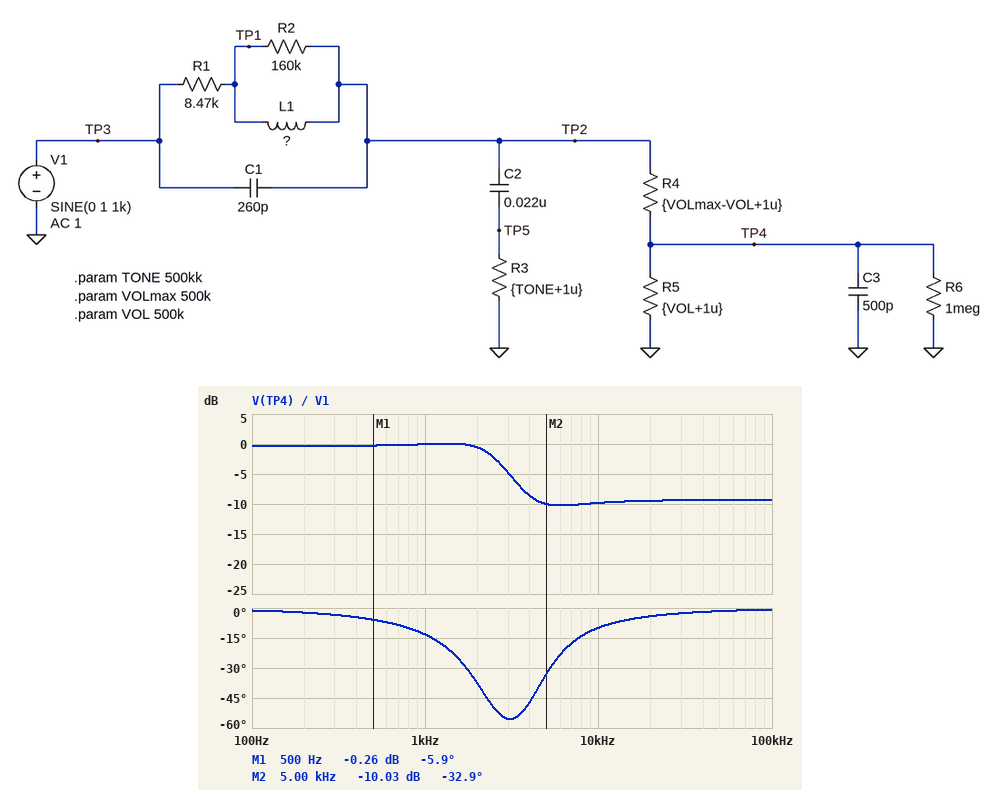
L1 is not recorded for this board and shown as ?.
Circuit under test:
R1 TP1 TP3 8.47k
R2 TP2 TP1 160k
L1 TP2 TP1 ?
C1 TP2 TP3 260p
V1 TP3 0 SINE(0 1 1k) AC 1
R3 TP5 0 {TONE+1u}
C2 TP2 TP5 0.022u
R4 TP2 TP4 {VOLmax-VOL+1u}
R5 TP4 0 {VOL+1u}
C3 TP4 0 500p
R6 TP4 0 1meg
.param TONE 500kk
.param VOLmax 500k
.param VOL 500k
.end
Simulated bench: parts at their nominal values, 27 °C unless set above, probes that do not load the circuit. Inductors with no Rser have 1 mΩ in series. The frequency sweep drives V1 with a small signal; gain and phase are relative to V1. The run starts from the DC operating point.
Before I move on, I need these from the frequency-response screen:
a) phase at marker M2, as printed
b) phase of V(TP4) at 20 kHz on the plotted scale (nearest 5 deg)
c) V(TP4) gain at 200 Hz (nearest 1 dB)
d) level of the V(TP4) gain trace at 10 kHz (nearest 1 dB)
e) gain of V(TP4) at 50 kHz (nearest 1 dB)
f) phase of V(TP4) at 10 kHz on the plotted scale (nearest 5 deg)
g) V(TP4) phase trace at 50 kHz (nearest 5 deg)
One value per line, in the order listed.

-32.9 deg
-5 deg
0 dB
-10 dB
-9 dB
-10 deg
0 deg
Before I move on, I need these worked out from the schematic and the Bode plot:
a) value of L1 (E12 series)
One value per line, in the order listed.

5.6 H
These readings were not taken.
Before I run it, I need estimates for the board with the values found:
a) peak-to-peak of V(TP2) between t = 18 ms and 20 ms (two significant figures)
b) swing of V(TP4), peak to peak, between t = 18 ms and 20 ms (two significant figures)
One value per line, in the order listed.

2.0 V
2.0 V
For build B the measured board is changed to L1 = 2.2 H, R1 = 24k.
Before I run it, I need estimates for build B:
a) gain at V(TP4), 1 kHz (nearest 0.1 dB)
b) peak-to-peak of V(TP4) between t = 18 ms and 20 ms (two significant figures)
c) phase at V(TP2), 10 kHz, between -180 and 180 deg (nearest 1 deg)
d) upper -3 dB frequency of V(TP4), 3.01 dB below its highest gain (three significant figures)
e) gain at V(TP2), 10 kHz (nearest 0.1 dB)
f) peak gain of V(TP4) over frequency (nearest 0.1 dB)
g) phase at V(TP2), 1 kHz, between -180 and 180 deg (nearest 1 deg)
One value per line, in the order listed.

-0.8 dB
1.8 V
-15 deg
4.07 kHz
-10.8 dB
-0.5 dB
-8 deg
